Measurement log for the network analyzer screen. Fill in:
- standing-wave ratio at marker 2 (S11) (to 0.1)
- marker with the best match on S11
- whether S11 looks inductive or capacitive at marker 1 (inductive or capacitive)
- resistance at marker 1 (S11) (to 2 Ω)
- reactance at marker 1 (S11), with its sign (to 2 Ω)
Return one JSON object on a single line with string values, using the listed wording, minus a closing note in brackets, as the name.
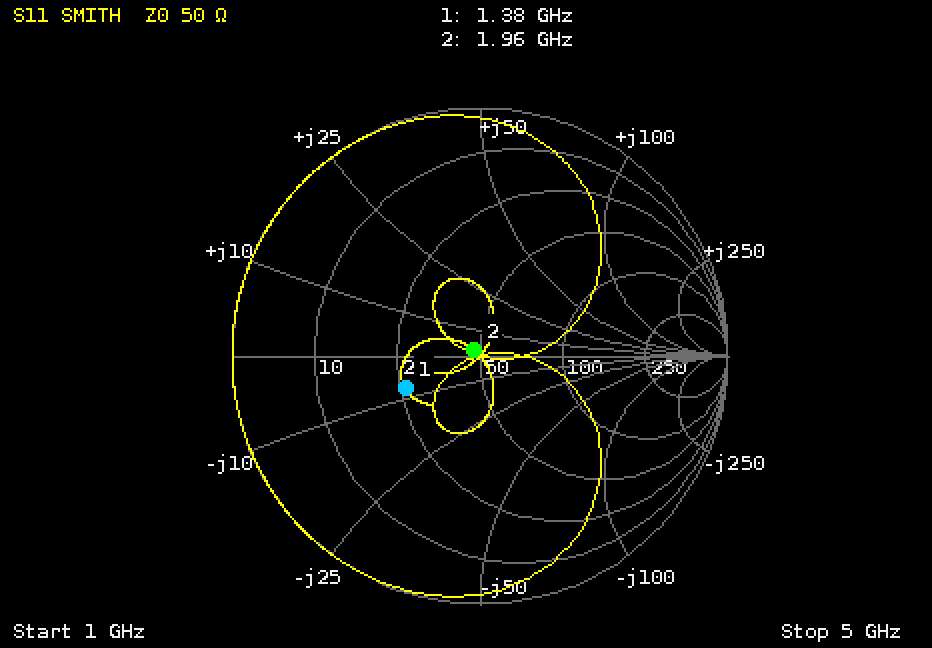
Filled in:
{"standing-wave ratio at marker 2 (S11)": "1.1", "marker with the best match on S11": "marker 2", "whether S11 looks inductive or capacitive at marker 1": "capacitive", "resistance at marker 1 (S11)": "26 Ω", "reactance at marker 1 (S11), with its sign": "-8 Ω"}
